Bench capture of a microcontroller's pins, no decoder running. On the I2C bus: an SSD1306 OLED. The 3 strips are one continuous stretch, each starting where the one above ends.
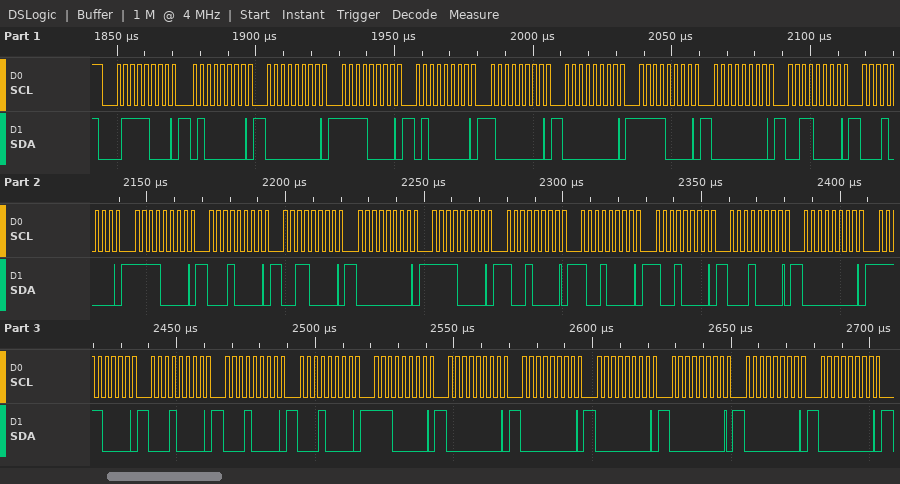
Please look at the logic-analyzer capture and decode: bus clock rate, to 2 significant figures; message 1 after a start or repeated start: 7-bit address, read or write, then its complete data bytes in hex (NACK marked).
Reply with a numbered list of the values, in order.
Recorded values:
1. 400 kHz
2. 0x3C write: 40 00 F0 40 80 00 F0 00 30 10 F0 10 30 00 F0 90 90 90 10 00 F0 10 10 10 E0 00 00 00 00 00 00
